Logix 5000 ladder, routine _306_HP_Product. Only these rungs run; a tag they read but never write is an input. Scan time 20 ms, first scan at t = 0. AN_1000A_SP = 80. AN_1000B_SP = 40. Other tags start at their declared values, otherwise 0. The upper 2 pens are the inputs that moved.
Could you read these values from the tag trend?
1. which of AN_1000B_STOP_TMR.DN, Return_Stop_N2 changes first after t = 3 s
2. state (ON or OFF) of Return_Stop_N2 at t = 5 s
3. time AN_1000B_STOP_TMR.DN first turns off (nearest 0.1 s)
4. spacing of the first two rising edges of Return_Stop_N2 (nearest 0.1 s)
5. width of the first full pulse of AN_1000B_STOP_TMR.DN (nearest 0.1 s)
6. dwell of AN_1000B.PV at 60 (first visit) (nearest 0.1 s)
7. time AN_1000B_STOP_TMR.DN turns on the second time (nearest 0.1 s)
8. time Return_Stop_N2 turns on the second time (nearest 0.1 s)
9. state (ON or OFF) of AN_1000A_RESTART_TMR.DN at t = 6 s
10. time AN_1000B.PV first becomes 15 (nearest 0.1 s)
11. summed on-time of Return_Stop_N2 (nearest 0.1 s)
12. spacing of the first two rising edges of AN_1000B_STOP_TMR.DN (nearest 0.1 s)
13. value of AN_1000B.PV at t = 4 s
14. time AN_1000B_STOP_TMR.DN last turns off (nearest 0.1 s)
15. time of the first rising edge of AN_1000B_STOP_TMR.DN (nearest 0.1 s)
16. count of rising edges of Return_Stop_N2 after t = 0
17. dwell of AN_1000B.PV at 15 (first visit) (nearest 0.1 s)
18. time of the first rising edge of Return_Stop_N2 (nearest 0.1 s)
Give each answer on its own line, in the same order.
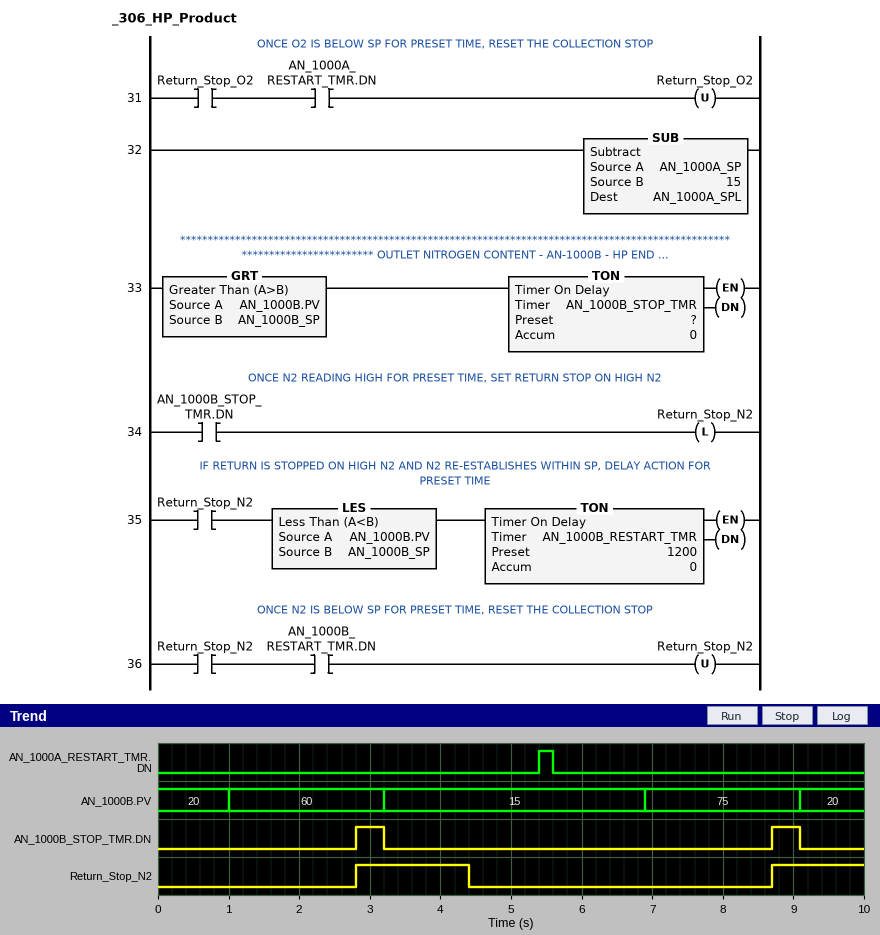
AN_1000B_STOP_TMR.DN
OFF
3.2 s
5.9 s
0.4 s
2.2 s
8.7 s
8.7 s
OFF
3.2 s
2.9 s
5.9 s
15
9.1 s
2.8 s
2
3.7 s
2.8 s
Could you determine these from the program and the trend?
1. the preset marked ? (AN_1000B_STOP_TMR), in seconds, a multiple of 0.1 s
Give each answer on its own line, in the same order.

1.8 s
